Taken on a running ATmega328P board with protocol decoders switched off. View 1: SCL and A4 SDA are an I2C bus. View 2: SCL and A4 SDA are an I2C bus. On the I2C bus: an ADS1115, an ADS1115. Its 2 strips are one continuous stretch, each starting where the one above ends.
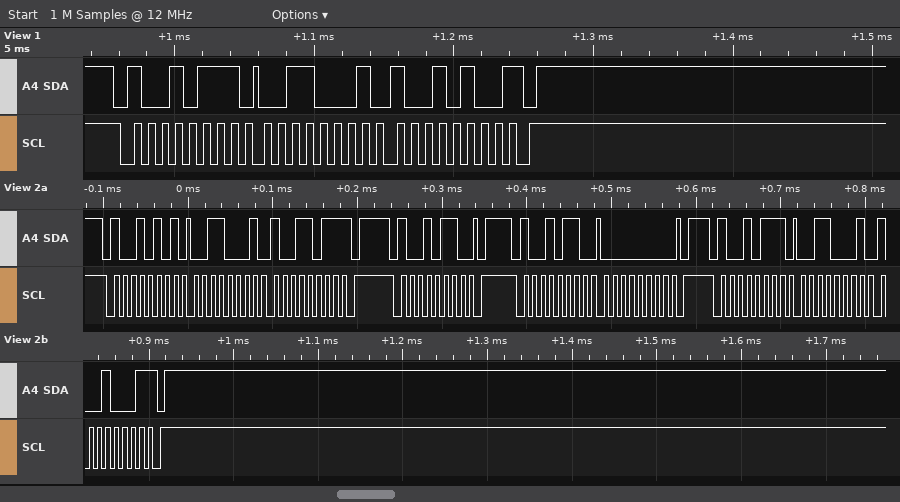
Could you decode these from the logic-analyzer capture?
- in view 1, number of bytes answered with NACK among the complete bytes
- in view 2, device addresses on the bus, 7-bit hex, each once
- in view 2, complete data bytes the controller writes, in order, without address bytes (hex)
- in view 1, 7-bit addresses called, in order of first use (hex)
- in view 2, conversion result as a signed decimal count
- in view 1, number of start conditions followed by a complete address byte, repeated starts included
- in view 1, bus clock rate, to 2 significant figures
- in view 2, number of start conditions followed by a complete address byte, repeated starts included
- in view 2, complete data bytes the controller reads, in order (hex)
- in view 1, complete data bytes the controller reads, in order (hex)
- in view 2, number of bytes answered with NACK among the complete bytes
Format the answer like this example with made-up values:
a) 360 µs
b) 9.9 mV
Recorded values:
a) 1
b) 0x4A 0x4B
c) 00
d) 0x4B
e) 12689
f) 1
g) 100 kHz
h) 4
i) 31 9B 31 91
j) 31 94
k) 2
